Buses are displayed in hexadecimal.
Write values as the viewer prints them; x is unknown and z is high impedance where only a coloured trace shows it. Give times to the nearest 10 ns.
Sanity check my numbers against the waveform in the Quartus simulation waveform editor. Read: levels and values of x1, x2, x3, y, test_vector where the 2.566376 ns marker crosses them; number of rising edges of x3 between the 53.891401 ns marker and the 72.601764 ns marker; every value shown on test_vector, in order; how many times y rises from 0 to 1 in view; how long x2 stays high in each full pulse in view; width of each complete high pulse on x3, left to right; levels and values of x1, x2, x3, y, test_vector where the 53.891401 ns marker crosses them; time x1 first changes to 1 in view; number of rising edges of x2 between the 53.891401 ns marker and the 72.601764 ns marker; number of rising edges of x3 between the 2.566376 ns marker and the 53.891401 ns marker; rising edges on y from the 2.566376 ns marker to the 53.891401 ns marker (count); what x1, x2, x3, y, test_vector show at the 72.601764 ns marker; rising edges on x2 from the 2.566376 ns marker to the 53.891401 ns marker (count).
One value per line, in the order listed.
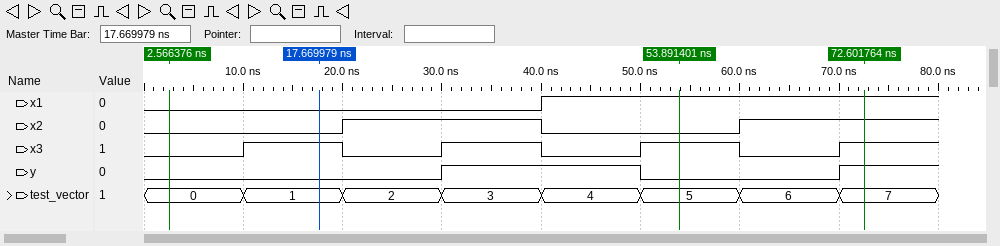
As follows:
x1=0, x2=0, x3=0, y=0, test_vector=0
1
0, 1, 2, 3, 4, 5, 6, 7
2
20 ns
10 ns, 10 ns, 10 ns
x1=1, x2=0, x3=1, y=0, test_vector=5
40 ns
1
3
1
x1=1, x2=1, x3=1, y=1, test_vector=7
1
